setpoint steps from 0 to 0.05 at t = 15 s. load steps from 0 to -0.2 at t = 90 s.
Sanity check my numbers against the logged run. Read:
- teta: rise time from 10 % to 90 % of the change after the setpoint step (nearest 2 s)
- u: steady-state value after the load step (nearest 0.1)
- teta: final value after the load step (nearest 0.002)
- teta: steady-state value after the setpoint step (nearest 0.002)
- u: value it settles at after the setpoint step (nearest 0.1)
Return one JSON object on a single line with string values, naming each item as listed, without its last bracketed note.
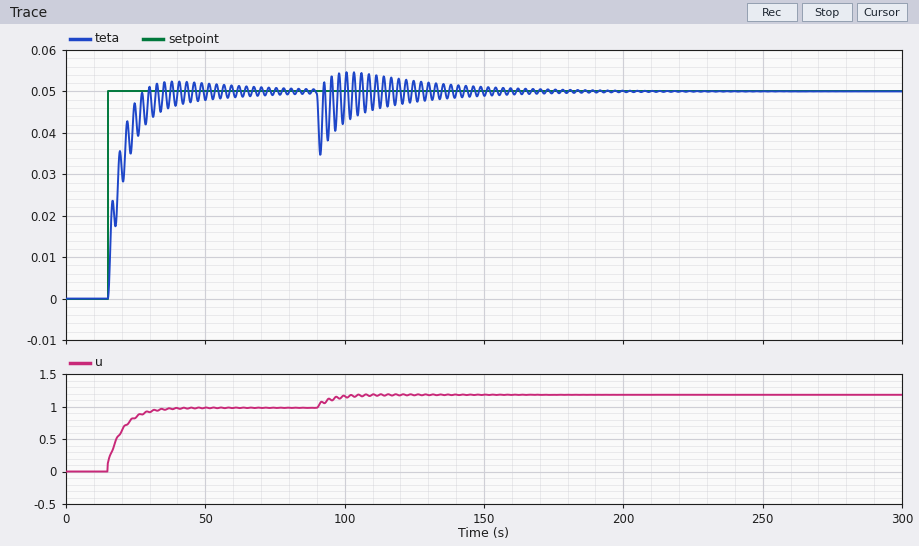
{"teta: rise time from 10 % to 90 % of the change after the setpoint step": "8 s", "u: steady-state value after the load step": "1.2", "teta: final value after the load step": "0.050", "teta: steady-state value after the setpoint step": "0.050", "u: value it settles at after the setpoint step": "1.0"}
